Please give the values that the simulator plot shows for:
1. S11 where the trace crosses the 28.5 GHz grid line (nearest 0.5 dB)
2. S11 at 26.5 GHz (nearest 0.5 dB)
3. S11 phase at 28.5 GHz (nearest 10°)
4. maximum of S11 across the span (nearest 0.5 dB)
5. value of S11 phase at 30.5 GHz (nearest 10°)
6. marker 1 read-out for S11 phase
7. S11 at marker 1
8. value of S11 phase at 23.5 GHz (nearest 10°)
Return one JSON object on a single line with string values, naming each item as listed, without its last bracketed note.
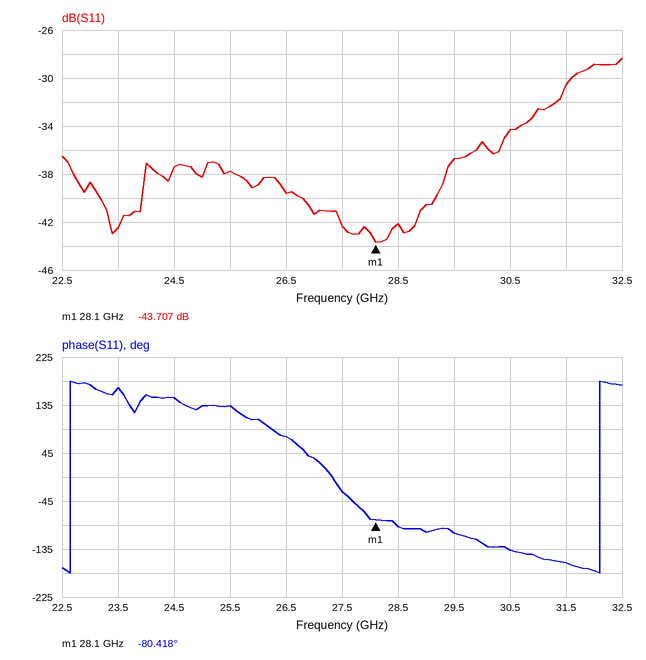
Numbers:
{"S11 where the trace crosses the 28.5 GHz grid line": "-42.0 dB", "S11 at 26.5 GHz": "-39.5 dB", "S11 phase at 28.5 GHz": "-90°", "maximum of S11 across the span": "-28.5 dB", "value of S11 phase at 30.5 GHz": "-140°", "marker 1 read-out for S11 phase": "-80.418°", "S11 at marker 1": "-43.707 dB", "value of S11 phase at 23.5 GHz": "170°"}
